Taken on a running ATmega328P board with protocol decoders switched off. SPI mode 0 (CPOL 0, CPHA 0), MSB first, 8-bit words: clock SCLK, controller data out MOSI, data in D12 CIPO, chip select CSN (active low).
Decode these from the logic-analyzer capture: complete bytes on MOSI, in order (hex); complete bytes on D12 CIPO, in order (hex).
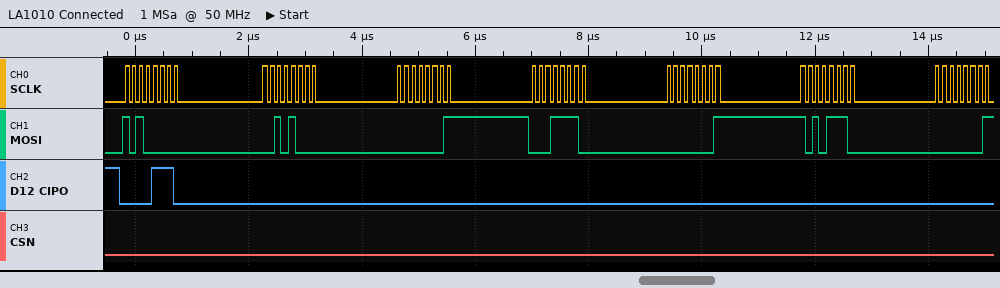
A0 28 01 1E 01 AE 01
0E 00 00 00 00 00 00
